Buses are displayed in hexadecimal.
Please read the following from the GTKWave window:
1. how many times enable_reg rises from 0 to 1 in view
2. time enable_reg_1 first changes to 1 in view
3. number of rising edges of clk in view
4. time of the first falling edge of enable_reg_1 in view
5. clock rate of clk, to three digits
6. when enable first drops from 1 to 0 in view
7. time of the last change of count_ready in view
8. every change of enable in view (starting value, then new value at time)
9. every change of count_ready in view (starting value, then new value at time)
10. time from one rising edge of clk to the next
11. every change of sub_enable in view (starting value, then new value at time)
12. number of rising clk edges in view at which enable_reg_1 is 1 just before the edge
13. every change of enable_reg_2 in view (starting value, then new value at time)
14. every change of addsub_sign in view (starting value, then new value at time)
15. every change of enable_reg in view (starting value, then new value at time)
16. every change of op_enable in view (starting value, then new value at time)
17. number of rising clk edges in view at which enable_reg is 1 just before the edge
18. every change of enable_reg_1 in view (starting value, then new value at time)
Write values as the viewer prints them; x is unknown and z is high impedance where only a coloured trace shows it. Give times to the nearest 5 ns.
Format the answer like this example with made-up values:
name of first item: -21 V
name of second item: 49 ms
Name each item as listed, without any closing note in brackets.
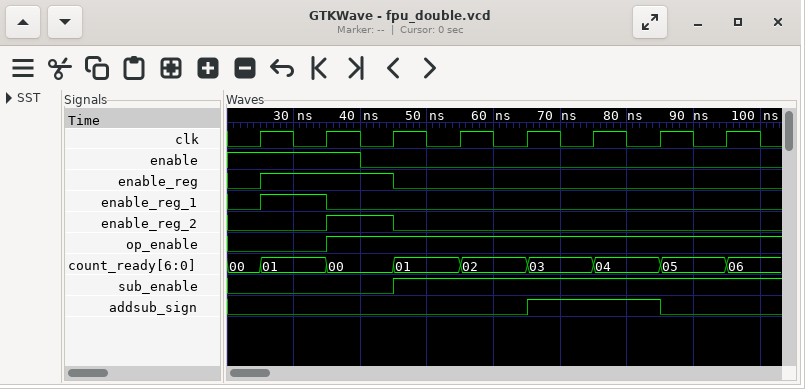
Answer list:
how many times enable_reg rises from 0 to 1 in view: 1
time enable_reg_1 first changes to 1 in view: 25 ns
number of rising edges of clk in view: 8
time of the first falling edge of enable_reg_1 in view: 35 ns
clock rate of clk, to three digits: 100 MHz
when enable first drops from 1 to 0 in view: 40 ns
time of the last change of count_ready in view: 95 ns
every change of enable in view: 1, 0 at 40 ns
every change of count_ready in view: 00, 01 at 25 ns, 00 at 35 ns, 01 at 45 ns, 02 at 55 ns, 03 at 65 ns, 04 at 75 ns, 05 at 85 ns, 06 at 95 ns
time from one rising edge of clk to the next: 10 ns
every change of sub_enable in view: 0, 1 at 45 ns
number of rising clk edges in view at which enable_reg_1 is 1 just before the edge: 1
every change of enable_reg_2 in view: 0, 1 at 35 ns, 0 at 45 ns
every change of addsub_sign in view: 0, 1 at 65 ns, 0 at 85 ns
every change of enable_reg in view: 0, 1 at 25 ns, 0 at 45 ns
every change of op_enable in view: 0, 1 at 35 ns
number of rising clk edges in view at which enable_reg is 1 just before the edge: 2
every change of enable_reg_1 in view: 0, 1 at 25 ns, 0 at 35 ns
